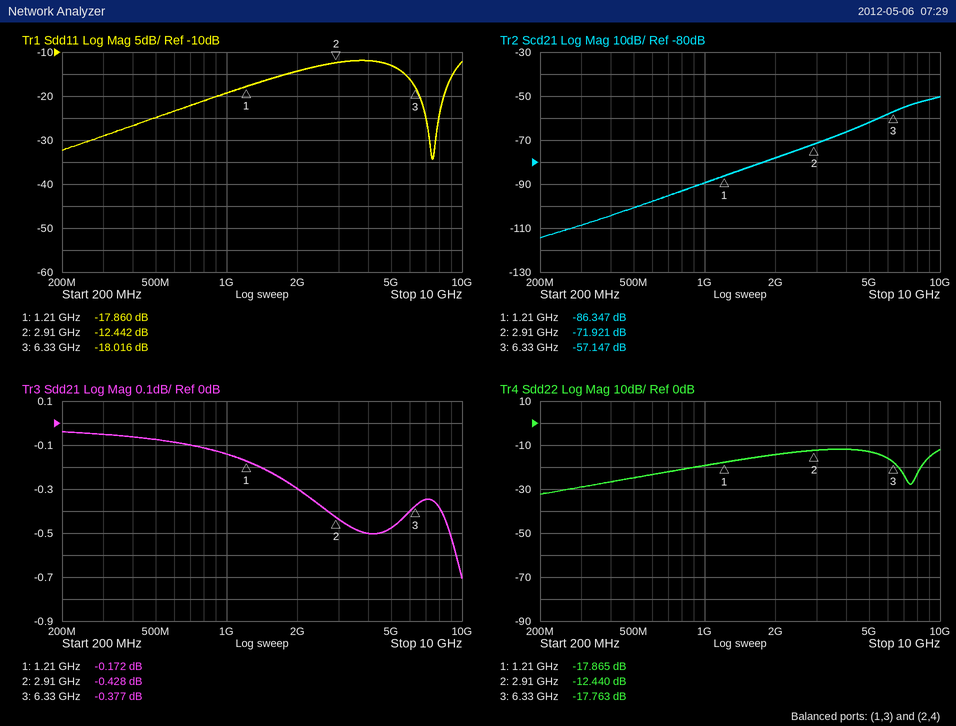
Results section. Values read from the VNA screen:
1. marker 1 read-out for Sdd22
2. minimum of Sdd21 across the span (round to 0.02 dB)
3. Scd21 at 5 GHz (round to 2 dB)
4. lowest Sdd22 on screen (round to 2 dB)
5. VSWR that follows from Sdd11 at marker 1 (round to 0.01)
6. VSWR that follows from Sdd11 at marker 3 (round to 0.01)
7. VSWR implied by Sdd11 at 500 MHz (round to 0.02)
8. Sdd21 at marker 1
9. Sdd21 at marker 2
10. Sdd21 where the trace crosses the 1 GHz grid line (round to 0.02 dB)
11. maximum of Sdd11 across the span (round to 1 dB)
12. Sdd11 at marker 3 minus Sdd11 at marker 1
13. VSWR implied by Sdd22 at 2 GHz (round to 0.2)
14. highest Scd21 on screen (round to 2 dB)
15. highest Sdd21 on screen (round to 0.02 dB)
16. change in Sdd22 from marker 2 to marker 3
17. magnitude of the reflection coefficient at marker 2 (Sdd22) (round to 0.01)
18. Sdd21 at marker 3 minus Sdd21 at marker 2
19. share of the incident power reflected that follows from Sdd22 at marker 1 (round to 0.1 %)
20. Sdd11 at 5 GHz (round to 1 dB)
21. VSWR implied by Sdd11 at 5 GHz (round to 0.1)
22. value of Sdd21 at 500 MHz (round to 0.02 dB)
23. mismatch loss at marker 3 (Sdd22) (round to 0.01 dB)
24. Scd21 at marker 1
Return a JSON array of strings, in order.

["-17.865 dB", "-0.70 dB", "-62 dB", "-32 dB", "1.29", "1.29", "1.12", "-0.172 dB", "-0.428 dB", "-0.14 dB", "-12 dB", "-0.156 dB", "1.4", "-50 dB", "-0.04 dB", "-5.323 dB", "0.24", "0.051 dB", "1.6 %", "-13 dB", "1.6", "-0.08 dB", "0.07 dB", "-86.347 dB"]
